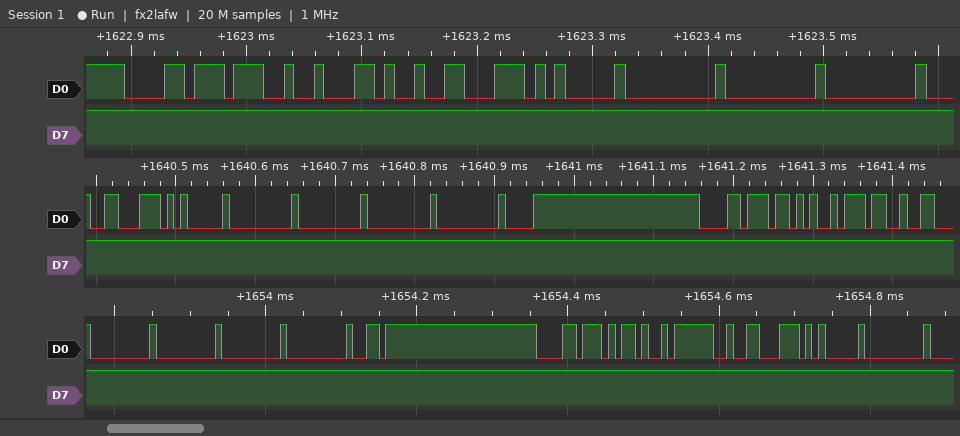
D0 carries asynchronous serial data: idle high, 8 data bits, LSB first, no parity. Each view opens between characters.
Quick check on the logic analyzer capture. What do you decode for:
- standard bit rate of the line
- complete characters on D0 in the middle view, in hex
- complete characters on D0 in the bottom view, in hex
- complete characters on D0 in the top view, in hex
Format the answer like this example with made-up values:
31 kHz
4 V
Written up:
115200 baud
C6, 05, 00, 00, 00, 00, F8, D8, 2B, 37
00, 00, 00, 00, F6, D8, 2D, 3F, C6, 05, 00
D8, 27, 2C, C6, 05, 00, 00, 00
